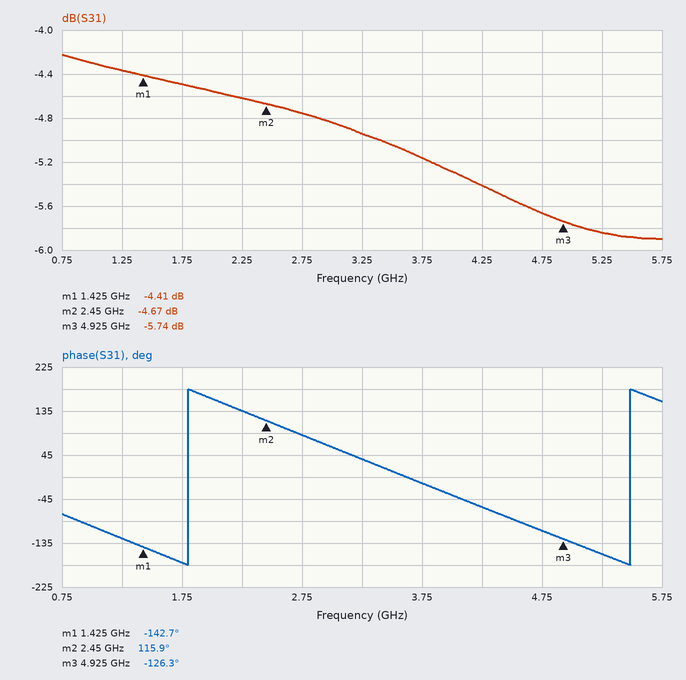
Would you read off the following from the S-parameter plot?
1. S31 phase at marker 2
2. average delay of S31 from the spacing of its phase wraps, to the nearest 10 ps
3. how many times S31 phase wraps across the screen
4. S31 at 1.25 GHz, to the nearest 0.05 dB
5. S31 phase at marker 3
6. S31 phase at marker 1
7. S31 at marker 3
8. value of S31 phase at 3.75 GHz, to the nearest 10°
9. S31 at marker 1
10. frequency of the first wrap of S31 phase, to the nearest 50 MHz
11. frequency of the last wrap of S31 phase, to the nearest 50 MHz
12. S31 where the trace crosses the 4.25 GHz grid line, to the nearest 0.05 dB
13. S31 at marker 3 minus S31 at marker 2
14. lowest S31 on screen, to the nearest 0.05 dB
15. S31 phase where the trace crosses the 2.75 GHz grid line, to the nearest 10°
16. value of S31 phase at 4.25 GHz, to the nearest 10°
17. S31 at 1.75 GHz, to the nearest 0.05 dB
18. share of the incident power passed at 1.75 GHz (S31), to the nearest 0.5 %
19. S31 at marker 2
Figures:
115.9°
270 ps
2
-4.35 dB
-126.3°
-142.7°
-5.74 dB
-10°
-4.41 dB
1.80 GHz
5.50 GHz
-5.40 dB
-1.07 dB
-5.90 dB
90°
-60°
-4.50 dB
35.5 %
-4.67 dB
